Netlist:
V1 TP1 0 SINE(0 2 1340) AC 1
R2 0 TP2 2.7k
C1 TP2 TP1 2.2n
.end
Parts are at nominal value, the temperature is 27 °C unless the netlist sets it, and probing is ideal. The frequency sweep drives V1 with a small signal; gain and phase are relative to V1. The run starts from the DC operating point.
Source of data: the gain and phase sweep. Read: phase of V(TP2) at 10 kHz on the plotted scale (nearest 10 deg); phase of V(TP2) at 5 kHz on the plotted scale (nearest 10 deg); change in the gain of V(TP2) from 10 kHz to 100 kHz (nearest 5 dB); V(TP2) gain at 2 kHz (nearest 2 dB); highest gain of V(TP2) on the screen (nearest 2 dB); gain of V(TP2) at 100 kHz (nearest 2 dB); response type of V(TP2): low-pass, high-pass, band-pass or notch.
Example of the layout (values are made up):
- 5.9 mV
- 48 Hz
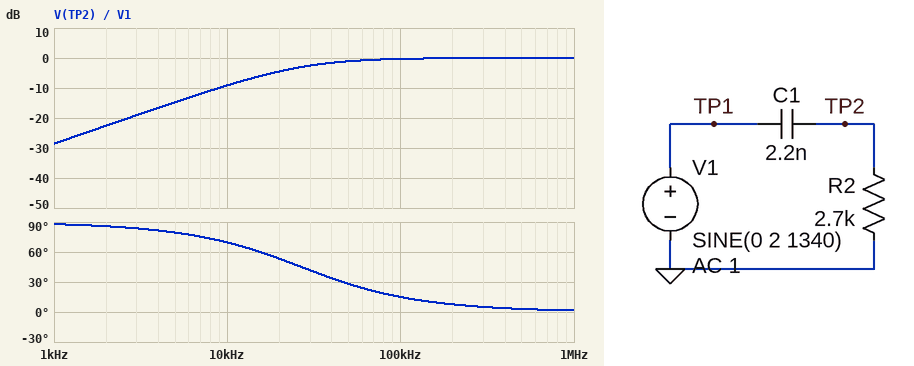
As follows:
- 70 deg
- 80 deg
- 10 dB
- -22 dB
- 0 dB
- 0 dB
- high-pass
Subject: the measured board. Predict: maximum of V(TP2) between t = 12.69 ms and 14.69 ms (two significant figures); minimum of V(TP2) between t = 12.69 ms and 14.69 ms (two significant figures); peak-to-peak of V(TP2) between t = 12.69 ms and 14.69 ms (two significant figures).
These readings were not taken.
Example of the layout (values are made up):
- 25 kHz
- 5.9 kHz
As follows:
- 100 mV
- -100 mV
- 200 mV
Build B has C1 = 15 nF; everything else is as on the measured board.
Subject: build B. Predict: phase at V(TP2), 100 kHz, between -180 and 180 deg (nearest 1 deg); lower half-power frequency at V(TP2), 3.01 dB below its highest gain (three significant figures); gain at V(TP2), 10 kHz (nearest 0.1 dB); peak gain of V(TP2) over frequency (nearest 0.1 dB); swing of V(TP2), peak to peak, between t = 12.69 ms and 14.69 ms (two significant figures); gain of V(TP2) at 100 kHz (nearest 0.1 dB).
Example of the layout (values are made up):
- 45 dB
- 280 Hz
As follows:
- 2 deg
- 3.93 kHz
- -0.6 dB
- 0 dB
- 1.3 V
- 0 dB
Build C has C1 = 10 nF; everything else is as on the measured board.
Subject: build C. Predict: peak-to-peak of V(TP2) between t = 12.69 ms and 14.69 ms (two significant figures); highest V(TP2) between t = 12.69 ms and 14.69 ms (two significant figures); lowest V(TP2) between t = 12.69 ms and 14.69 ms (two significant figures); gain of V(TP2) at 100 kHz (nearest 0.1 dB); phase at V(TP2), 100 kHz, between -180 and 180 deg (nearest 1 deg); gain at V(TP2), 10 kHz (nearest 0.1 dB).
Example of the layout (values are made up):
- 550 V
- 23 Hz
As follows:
- 890 mV
- 440 mV
- -440 mV
- 0 dB
- 3 deg
- -1.3 dB
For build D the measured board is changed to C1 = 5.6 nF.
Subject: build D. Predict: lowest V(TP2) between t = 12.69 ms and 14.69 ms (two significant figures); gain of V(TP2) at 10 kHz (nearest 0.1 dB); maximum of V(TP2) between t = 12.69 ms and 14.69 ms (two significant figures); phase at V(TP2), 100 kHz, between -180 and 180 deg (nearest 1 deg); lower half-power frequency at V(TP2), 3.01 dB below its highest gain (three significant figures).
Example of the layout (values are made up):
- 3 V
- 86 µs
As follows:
- -250 mV
- -3.2 dB
- 250 mV
- 6 deg
- 10.5 kHz
